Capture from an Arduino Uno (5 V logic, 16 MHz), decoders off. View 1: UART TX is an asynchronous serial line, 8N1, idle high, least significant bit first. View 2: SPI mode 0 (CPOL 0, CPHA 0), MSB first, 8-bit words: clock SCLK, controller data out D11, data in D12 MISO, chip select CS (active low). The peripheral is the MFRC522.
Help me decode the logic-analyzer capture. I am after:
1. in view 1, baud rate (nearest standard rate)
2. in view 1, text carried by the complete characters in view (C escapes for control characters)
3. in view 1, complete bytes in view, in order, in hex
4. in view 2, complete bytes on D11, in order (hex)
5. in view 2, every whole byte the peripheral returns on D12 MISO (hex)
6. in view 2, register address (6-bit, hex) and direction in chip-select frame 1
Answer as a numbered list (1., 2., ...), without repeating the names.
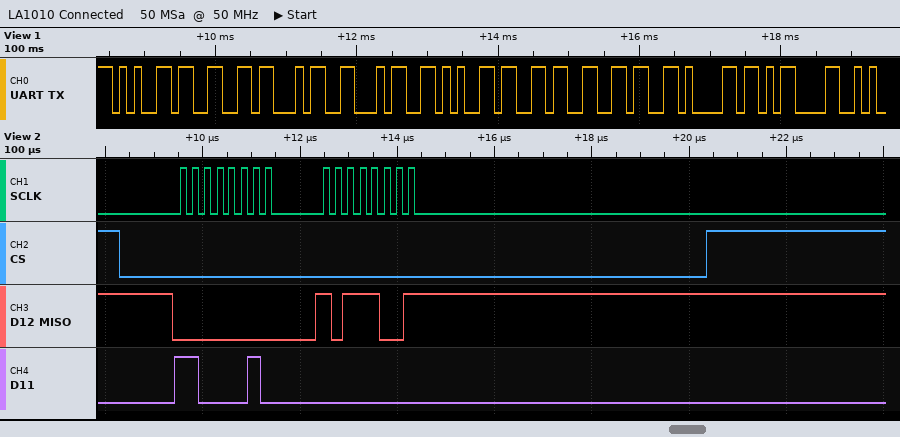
1. 9600 baud
2. "ef44e66a\r"
3. 65 66 34 34 65 36 36 61 0D
4. C2 00
5. 00 B9
6. 0x21 read
